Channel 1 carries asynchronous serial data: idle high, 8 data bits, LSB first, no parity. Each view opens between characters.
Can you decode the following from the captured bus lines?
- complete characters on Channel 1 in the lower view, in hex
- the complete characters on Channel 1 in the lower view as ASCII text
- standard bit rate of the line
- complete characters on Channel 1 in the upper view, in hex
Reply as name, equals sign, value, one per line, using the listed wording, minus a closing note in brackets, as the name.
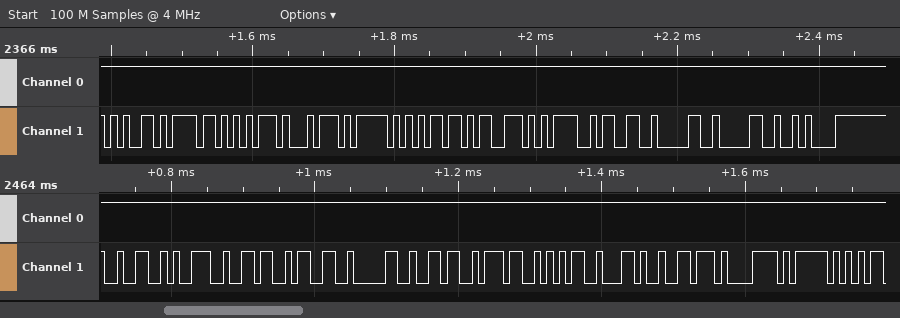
complete characters on Channel 1 in the lower view, in hex = 32, 39, 36, 33, 30, 36, 37, 35, 2C, 76, 78, 5F
the complete characters on Channel 1 in the lower view as ASCII text = "29630675,vx_"
standard bit rate of the line = 115200 baud
complete characters on Channel 1 in the upper view, in hex = 65, 6F, 75, 74, 5F, 6D, 73, 3D, 33, 30, 30, 0A
